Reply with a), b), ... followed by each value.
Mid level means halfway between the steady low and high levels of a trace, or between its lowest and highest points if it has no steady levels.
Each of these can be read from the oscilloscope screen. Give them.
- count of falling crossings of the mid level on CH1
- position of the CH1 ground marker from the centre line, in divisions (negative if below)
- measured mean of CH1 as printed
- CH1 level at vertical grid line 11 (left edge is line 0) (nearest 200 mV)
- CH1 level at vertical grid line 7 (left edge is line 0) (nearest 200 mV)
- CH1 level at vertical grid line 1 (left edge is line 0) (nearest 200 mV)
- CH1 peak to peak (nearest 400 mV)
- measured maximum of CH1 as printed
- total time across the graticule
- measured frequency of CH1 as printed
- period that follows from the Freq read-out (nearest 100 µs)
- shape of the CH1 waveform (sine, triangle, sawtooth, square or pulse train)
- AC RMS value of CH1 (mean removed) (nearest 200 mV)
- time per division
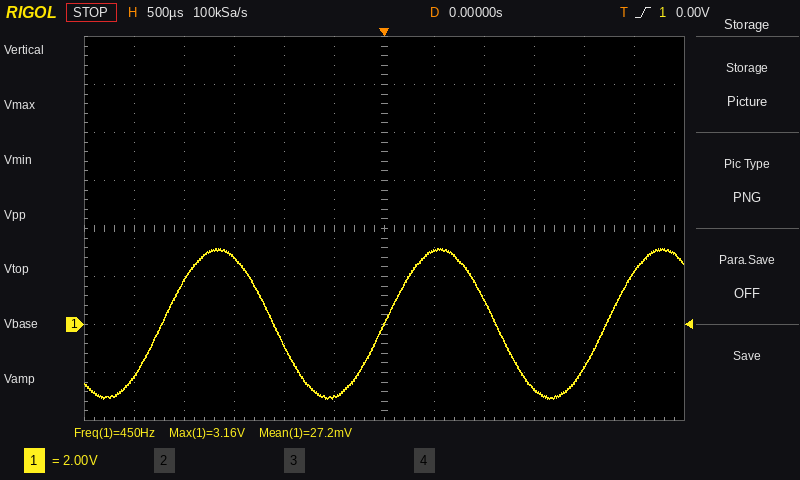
a) 2
b) -2.0 div
c) 27.2 mV
d) 2.2 V
e) 3.0 V
f) -2.2 V
g) 6.4 V
h) 3.16 V
i) 6 ms
j) 450 Hz
k) 2.2 ms
l) sine
m) 2.2 V
n) 500 µs
